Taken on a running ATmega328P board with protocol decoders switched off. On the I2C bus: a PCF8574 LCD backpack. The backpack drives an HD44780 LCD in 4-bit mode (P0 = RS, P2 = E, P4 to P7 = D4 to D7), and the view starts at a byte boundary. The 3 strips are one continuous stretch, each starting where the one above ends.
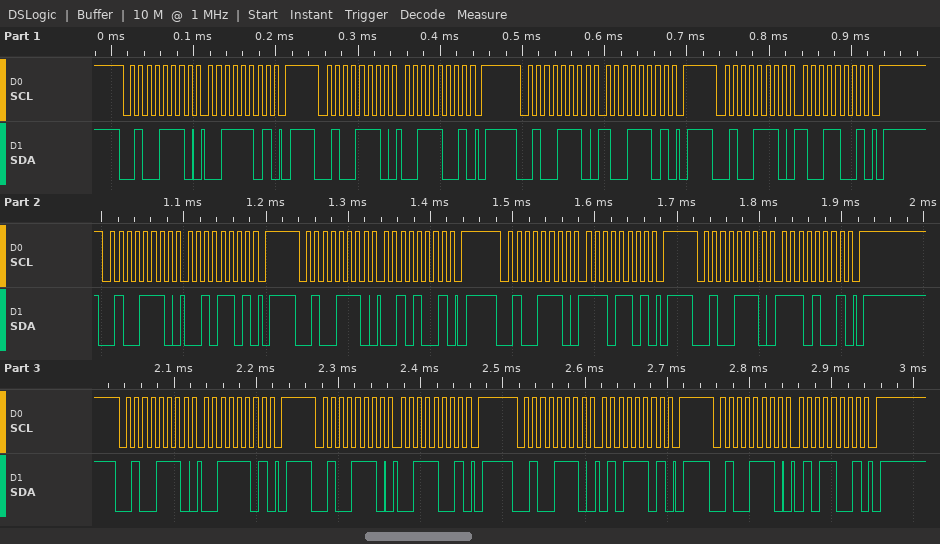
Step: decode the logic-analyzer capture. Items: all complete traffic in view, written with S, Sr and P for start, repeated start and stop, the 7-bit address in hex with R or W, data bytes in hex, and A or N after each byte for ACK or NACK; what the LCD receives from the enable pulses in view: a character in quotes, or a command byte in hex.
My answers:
S 27W A 3D A P S 27W A 39 A P S 27W A 9D A P S 27W A 99 A P S 27W A 2D A P S 27W A 29 A P S 27W A ED A P S 27W A E9 A P S 27W A 3D A P S 27W A 39 A P S 27W A 5D A P S 27W A 59 A P
'9' '.' '5'
